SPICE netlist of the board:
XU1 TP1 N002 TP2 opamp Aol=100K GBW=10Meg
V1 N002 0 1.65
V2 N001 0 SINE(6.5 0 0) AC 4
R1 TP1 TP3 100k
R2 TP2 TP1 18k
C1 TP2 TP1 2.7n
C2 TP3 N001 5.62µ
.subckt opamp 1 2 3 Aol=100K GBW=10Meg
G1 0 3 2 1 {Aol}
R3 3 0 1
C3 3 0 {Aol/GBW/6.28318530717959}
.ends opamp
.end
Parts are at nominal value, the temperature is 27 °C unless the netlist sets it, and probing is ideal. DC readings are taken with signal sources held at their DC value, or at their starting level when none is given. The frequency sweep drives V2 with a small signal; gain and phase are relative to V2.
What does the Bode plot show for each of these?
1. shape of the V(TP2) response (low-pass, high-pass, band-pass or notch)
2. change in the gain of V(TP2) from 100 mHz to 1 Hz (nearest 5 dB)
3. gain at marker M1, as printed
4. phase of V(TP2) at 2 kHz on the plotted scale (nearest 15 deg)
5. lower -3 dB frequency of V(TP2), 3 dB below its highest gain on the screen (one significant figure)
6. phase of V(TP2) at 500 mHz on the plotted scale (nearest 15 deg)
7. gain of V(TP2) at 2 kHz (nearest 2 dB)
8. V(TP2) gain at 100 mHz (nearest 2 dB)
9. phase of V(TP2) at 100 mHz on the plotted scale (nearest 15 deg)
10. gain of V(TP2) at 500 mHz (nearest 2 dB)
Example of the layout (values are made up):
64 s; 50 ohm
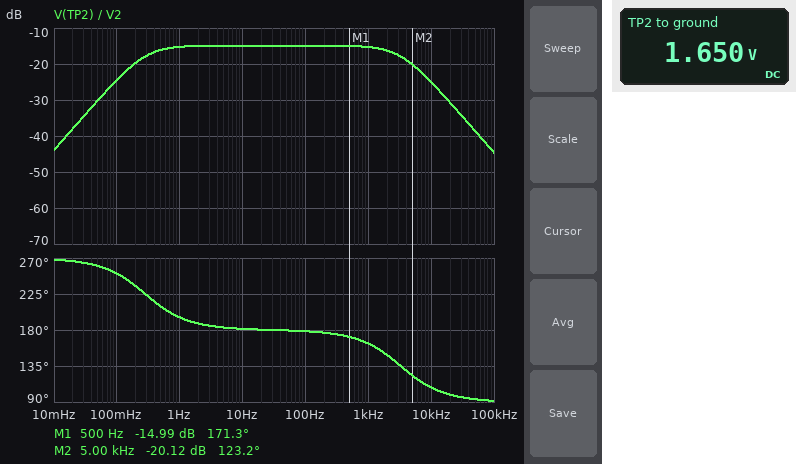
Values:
band-pass; 10 dB; -14.99 dB; 150 deg; 300 mHz; 210 deg; -16 dB; -24 dB; 255 deg; -16 dB
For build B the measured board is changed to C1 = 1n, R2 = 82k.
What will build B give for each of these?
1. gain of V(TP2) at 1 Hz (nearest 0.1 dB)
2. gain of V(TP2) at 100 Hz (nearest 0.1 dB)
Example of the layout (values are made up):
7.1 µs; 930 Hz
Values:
-2.1 dB; -1.7 dB
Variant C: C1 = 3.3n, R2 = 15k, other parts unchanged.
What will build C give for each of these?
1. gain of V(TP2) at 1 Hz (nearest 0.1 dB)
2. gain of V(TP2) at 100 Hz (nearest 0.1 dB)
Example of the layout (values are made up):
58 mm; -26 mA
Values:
-16.8 dB; -16.5 dB
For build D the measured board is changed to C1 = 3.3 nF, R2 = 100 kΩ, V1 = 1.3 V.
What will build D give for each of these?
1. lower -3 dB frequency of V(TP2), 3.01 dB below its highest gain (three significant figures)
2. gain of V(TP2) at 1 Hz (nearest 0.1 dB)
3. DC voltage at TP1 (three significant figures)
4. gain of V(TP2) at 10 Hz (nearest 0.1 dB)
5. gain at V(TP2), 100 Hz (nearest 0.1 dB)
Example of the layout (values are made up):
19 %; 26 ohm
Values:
283 mHz; -0.3 dB; 1.30 V; 0 dB; -0.2 dB
